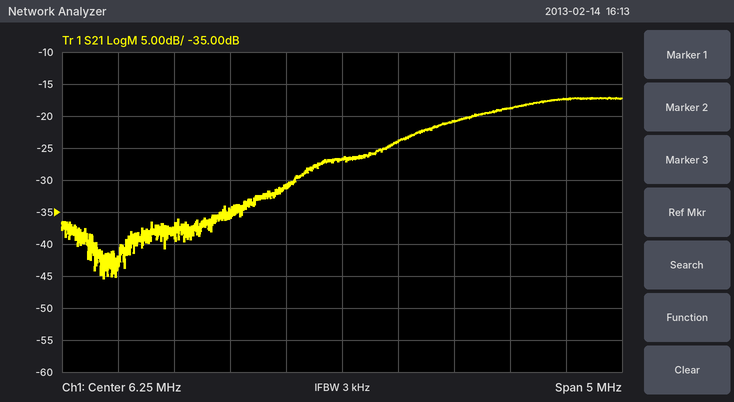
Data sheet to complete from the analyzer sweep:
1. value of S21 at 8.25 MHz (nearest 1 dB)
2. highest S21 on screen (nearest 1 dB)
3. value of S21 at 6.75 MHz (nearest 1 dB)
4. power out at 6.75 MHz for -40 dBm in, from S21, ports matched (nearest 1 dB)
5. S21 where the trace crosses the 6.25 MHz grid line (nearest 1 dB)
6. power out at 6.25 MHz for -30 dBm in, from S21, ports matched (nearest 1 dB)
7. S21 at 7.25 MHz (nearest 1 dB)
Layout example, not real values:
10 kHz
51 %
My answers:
-17 dB
-17 dB
-24 dB
-64 dBm
-27 dB
-57 dBm
-21 dB
